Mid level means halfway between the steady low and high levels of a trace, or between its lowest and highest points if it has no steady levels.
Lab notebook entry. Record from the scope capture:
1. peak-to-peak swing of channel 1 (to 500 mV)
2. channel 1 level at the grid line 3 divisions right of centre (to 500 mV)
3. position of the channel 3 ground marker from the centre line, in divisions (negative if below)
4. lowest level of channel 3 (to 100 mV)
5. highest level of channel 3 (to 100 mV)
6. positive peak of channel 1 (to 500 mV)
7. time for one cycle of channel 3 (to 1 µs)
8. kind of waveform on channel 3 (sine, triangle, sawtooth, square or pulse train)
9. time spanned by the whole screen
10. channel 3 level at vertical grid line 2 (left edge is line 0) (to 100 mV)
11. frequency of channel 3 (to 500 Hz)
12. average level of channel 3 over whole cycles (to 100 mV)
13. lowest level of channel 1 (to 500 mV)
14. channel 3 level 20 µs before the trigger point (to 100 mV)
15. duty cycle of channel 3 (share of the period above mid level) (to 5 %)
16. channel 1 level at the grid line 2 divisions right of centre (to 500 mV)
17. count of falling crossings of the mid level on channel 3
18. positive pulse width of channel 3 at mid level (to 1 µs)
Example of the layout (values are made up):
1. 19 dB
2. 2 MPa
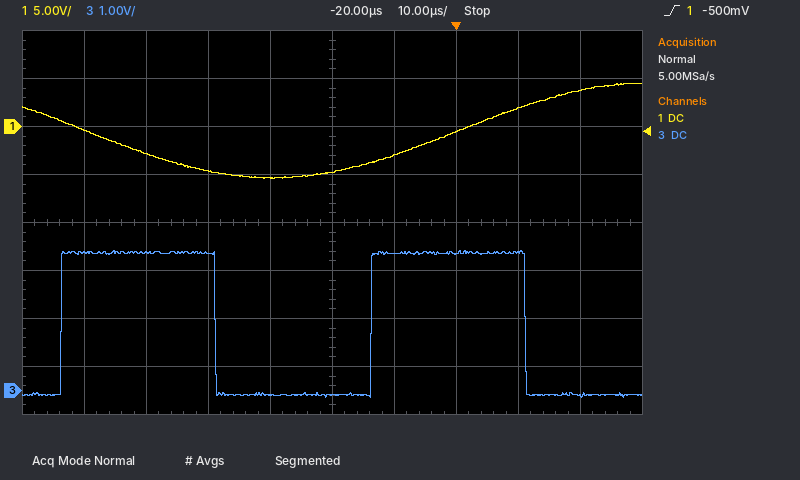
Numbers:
1. 10.0 V
2. 2.0 V
3. -3.5 div
4. -100 mV
5. 2.9 V
6. 4.5 V
7. 50 µs
8. square
9. 100 µs
10. 2.9 V
11. 20.0 kHz
12. 1.4 V
13. -5.5 V
14. -100 mV
15. 50 %
16. -500 mV
17. 2
18. 25 µs
